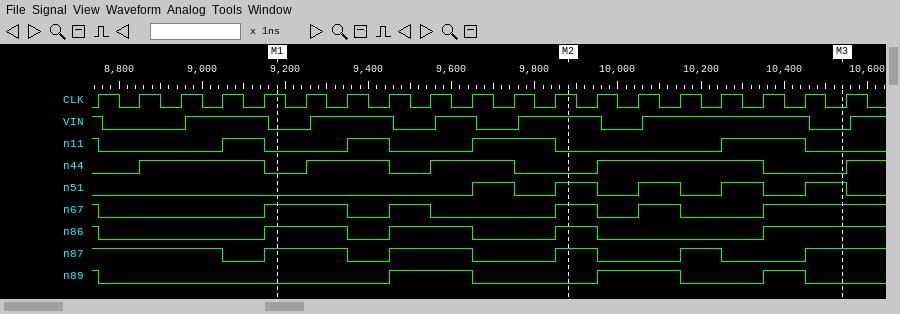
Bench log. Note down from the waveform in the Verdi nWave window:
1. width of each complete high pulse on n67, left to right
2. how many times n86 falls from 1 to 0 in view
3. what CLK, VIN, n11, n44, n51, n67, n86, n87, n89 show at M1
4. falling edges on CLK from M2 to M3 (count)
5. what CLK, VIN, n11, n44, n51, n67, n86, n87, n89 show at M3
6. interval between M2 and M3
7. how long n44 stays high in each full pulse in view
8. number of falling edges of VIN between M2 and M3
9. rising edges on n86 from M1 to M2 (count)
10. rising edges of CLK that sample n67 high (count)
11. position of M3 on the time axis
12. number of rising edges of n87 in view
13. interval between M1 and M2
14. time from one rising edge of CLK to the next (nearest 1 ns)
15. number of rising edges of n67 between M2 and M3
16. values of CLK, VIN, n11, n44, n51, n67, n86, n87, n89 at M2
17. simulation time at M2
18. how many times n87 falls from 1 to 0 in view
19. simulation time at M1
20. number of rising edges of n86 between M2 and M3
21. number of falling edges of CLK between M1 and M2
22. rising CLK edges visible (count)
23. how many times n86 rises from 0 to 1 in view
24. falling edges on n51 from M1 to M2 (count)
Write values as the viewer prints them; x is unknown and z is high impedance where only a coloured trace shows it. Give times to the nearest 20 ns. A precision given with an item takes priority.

200 ns, 100 ns, 100 ns, 100 ns
4
CLK=1, VIN=0, n11=0, n44=0, n51=0, n67=1, n86=1, n87=1, n89=0
7
CLK=0, VIN=0, n11=0, n44=0, n51=1, n67=1, n86=1, n87=1, n89=0
660 ns
300 ns, 200 ns, 200 ns, 400 ns
2
2
8
10540 ns
5
700 ns
100 ns
2
CLK=1, VIN=1, n11=0, n44=0, n51=1, n67=1, n86=1, n87=1, n89=0
9880 ns
5
9180 ns
1
7
19
4
1
